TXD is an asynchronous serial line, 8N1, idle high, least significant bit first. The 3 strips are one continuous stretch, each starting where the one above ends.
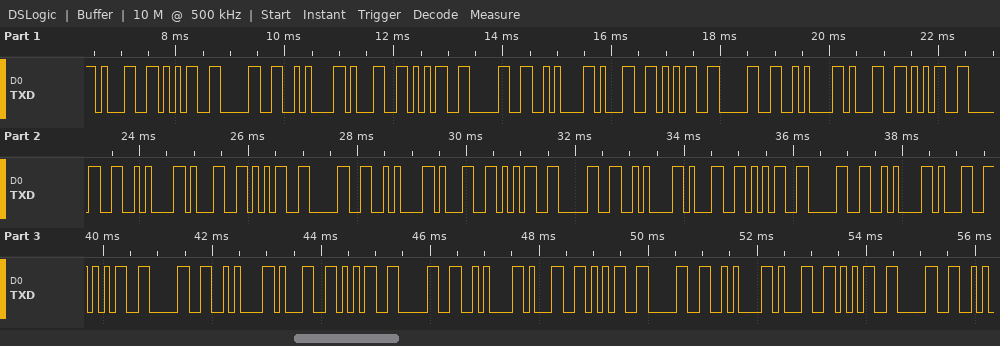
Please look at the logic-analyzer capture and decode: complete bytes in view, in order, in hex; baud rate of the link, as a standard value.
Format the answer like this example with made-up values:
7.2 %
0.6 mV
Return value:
31 35 30 0A 31 35 30 0A 31 35 30 0A 31 35 30 0A 31 35 30 0A 31 35 30 0A 31 35 30 0A 31 35 30 0A 31 35 30 0A 31 35 30 0A 31 35 30
9600 baud
